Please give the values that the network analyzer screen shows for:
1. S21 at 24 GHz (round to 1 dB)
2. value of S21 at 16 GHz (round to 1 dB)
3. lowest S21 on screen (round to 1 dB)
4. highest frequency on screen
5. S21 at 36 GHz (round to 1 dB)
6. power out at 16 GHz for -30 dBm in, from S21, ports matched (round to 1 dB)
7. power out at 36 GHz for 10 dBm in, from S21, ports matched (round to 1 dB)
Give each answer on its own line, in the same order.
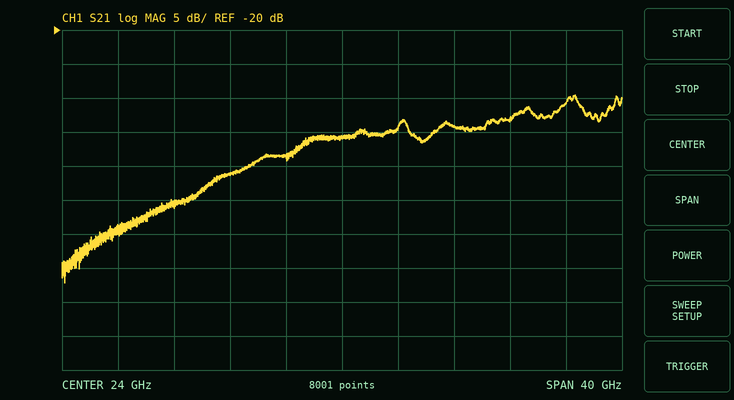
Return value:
-36 dB
-41 dB
-57 dB
44 GHz
-33 dB
-71 dBm
-23 dBm
